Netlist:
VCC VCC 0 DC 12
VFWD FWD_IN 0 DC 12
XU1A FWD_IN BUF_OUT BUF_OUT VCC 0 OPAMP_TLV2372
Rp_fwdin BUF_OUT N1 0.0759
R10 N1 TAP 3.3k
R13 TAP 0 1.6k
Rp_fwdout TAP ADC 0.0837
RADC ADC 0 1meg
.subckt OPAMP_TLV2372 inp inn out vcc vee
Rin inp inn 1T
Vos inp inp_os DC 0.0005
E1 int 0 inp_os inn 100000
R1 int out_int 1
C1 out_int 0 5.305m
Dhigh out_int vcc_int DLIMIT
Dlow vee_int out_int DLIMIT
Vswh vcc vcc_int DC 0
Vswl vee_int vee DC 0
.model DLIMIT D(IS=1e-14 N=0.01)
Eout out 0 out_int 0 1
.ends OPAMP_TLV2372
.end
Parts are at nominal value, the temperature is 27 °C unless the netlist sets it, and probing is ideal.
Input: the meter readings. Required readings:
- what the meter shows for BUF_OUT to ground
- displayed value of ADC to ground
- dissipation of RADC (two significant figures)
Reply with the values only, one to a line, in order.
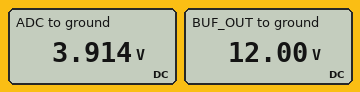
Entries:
12.00 V
3.914 V
15 µW
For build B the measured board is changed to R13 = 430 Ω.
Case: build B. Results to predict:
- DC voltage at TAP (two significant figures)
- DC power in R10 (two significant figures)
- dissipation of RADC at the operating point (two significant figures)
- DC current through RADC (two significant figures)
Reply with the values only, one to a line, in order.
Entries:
1.4 V
34 mW
1.9 µW
1.4 µA
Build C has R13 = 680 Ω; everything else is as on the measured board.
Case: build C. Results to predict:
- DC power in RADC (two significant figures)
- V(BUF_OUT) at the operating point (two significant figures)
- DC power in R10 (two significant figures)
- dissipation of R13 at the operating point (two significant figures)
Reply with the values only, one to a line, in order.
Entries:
4.2 µW
12 V
30 mW
6.2 mW
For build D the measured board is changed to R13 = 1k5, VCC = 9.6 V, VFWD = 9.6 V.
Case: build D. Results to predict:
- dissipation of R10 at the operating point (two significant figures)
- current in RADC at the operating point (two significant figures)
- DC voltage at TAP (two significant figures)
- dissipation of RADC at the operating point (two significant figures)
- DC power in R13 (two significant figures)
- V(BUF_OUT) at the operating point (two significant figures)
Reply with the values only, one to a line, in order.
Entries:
13 mW
3.0 µA
3.0 V
9.0 µW
6.0 mW
9.6 V
